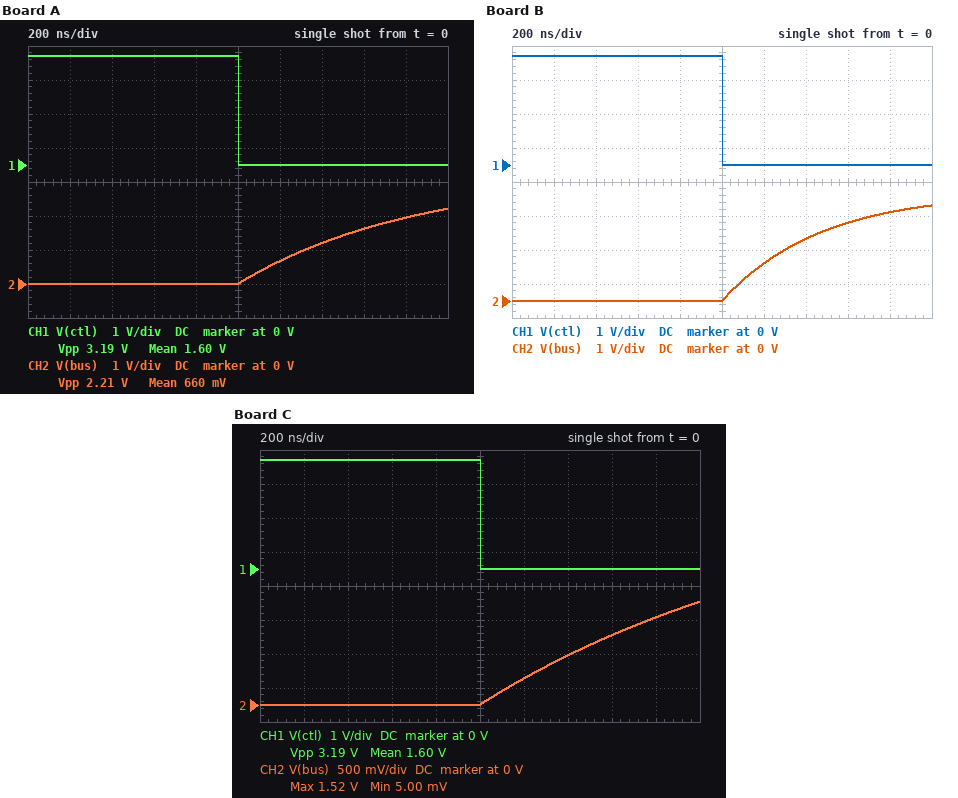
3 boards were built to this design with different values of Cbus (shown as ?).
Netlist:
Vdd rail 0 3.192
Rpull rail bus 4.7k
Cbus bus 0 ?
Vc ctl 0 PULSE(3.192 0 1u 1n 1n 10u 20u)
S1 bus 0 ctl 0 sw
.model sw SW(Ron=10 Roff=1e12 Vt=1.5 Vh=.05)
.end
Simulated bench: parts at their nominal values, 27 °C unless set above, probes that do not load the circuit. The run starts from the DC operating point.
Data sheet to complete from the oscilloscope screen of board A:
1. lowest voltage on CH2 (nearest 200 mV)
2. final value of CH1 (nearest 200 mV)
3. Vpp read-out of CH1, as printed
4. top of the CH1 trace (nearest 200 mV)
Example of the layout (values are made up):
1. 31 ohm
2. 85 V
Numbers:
1. 0 V
2. 0 V
3. 3.19 V
4. 3.2 V
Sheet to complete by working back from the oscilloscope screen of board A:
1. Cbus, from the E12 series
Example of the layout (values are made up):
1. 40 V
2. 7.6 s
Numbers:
1. 180 pF
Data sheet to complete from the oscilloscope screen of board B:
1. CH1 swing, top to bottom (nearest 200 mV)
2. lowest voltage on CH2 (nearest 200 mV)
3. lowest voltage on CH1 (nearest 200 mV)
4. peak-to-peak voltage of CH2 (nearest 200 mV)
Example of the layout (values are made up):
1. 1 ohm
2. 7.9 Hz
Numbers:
1. 3.2 V
2. 0 V
3. 0 V
4. 2.8 V
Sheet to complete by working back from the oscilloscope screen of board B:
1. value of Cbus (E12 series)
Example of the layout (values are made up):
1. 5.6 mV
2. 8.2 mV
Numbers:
1. 100 pF
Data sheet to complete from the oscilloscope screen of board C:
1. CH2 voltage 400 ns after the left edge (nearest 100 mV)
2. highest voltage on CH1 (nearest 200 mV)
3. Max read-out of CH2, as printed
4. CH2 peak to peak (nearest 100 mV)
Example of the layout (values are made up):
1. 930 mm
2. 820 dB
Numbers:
1. 0 V
2. 3.2 V
3. 1.52 V
4. 1.5 V
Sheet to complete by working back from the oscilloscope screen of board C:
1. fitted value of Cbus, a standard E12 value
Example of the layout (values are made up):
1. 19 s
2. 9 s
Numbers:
1. 330 pF
